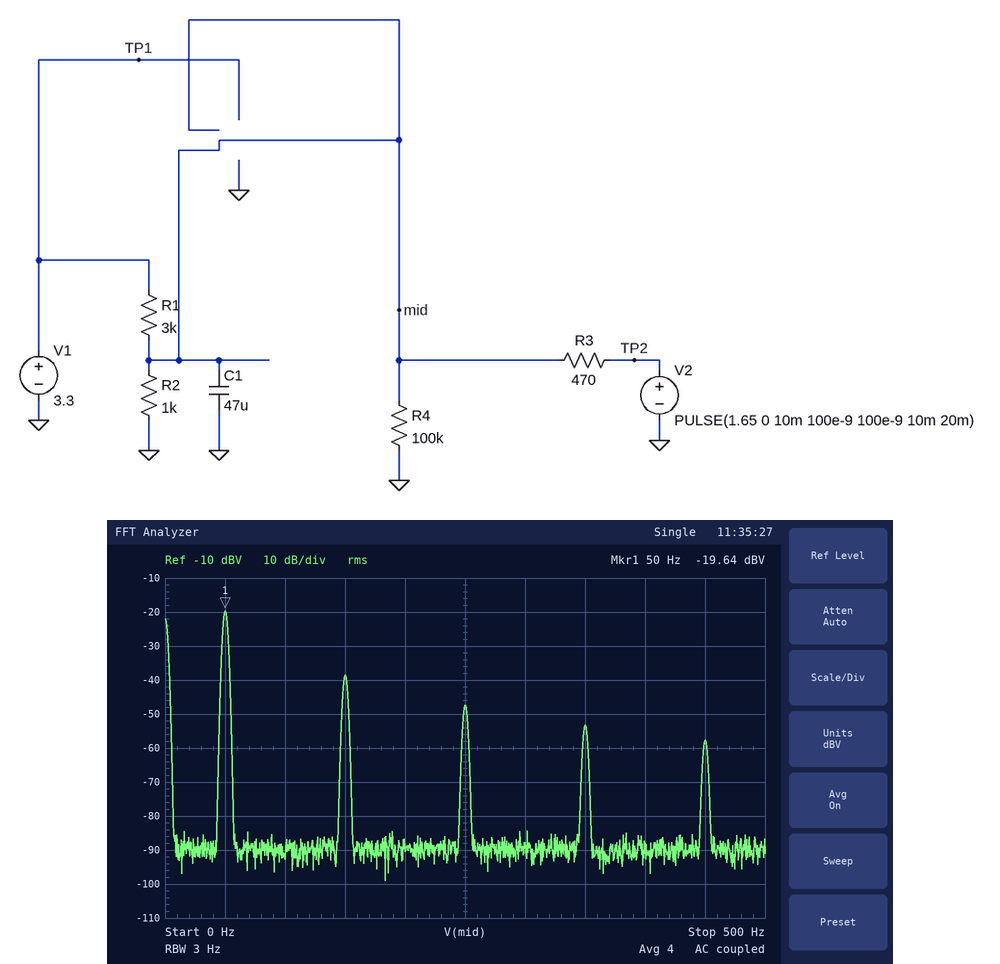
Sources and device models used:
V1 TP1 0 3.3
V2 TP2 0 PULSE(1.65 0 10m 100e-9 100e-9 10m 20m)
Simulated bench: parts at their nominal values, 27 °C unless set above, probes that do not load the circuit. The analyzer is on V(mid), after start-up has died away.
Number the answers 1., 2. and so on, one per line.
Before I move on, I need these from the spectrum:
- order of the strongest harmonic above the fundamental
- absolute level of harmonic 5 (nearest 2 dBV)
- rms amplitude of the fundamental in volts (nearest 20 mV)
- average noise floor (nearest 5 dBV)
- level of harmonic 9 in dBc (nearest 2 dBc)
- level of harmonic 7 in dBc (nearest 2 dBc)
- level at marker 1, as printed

1. 3
2. -48 dBV
3. 100 mV
4. -90 dBV
5. -38 dBc
6. -34 dBc
7. -19.64 dBV
